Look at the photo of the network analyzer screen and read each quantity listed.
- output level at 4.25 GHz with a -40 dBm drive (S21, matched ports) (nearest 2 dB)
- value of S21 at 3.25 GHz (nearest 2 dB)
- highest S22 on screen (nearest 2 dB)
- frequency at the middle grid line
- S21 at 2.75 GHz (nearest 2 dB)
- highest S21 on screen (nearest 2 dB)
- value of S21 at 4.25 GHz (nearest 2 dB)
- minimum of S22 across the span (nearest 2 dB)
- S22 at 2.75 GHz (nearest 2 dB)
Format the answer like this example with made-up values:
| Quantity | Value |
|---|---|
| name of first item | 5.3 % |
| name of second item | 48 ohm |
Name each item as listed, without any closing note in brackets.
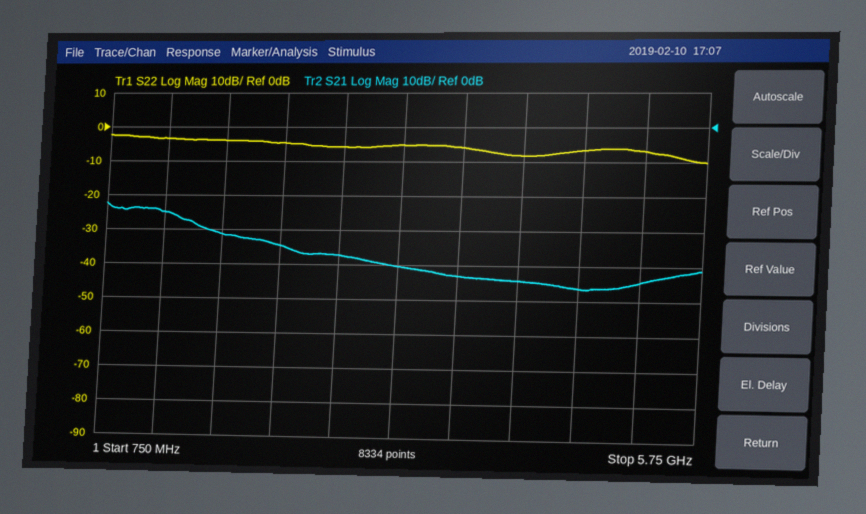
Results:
| Quantity | Value |
|---|---|
| output level at 4.25 GHz with a -40 dBm drive (S21, matched ports) | -84 dBm |
| value of S21 at 3.25 GHz | -40 dB |
| highest S22 on screen | -2 dB |
| frequency at the middle grid line | 3.25 GHz |
| S21 at 2.75 GHz | -38 dB |
| highest S21 on screen | -22 dB |
| value of S21 at 4.25 GHz | -44 dB |
| minimum of S22 across the span | -10 dB |
| S22 at 2.75 GHz | -6 dB |
